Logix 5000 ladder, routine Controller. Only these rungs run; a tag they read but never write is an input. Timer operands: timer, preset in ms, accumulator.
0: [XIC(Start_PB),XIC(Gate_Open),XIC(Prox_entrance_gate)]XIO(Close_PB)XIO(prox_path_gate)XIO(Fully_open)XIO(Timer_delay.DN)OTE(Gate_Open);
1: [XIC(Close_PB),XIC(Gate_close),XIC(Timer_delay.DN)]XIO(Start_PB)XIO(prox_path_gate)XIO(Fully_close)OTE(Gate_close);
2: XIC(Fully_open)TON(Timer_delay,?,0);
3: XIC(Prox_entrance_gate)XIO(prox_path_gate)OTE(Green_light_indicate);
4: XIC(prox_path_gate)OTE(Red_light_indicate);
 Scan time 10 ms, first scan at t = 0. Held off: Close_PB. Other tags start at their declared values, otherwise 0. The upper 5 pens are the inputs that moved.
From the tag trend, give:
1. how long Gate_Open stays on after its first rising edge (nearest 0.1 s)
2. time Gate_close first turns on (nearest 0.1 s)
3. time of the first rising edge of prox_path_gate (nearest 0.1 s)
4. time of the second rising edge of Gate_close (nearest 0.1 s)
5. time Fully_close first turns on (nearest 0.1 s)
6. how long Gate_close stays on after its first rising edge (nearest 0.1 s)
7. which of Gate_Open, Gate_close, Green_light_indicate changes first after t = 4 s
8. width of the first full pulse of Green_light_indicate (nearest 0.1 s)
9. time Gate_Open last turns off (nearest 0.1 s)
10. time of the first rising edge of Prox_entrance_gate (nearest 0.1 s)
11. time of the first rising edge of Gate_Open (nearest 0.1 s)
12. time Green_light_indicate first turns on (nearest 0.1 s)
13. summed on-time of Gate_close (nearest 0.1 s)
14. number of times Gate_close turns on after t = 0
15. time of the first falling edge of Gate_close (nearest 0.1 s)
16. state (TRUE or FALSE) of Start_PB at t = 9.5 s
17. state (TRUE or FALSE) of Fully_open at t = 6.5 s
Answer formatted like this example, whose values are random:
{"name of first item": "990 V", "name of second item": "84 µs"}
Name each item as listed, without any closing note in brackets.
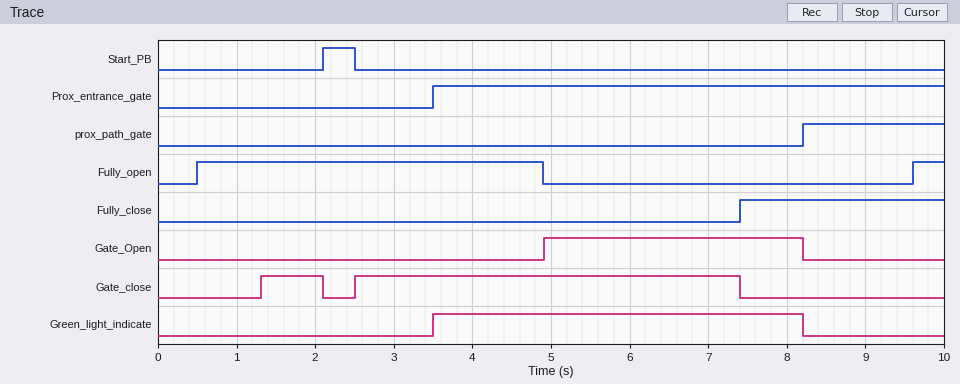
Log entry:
{"how long Gate_Open stays on after its first rising edge": "3.3 s", "time Gate_close first turns on": "1.3 s", "time of the first rising edge of prox_path_gate": "8.2 s", "time of the second rising edge of Gate_close": "2.5 s", "time Fully_close first turns on": "7.4 s", "how long Gate_close stays on after its first rising edge": "0.8 s", "which of Gate_Open, Gate_close, Green_light_indicate changes first after t = 4 s": "Gate_Open", "width of the first full pulse of Green_light_indicate": "4.7 s", "time Gate_Open last turns off": "8.2 s", "time of the first rising edge of Prox_entrance_gate": "3.5 s", "time of the first rising edge of Gate_Open": "4.9 s", "time Green_light_indicate first turns on": "3.5 s", "summed on-time of Gate_close": "5.7 s", "number of times Gate_close turns on after t = 0": "2", "time of the first falling edge of Gate_close": "2.1 s", "state (TRUE or FALSE) of Start_PB at t = 9.5 s": "FALSE", "state (TRUE or FALSE) of Fully_open at t = 6.5 s": "FALSE"}
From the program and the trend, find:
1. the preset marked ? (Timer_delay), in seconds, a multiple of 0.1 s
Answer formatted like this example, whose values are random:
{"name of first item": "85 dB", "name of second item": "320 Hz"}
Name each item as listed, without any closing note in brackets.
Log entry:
{"the preset marked ? (Timer_delay), in seconds, a multiple of 0.1 s": "0.8 s"}
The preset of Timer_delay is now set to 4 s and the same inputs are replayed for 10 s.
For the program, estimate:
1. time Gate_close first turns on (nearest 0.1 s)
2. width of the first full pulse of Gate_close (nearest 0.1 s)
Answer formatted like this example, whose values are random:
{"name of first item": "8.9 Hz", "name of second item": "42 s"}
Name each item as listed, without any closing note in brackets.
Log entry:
{"time Gate_close first turns on": "4.5 s", "width of the first full pulse of Gate_close": "2.9 s"}
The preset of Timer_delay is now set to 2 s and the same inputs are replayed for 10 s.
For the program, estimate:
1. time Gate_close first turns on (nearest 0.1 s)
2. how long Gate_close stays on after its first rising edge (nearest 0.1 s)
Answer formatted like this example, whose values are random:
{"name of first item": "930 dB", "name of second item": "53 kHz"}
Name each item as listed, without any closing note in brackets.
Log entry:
{"time Gate_close first turns on": "2.5 s", "how long Gate_close stays on after its first rising edge": "4.9 s"}
